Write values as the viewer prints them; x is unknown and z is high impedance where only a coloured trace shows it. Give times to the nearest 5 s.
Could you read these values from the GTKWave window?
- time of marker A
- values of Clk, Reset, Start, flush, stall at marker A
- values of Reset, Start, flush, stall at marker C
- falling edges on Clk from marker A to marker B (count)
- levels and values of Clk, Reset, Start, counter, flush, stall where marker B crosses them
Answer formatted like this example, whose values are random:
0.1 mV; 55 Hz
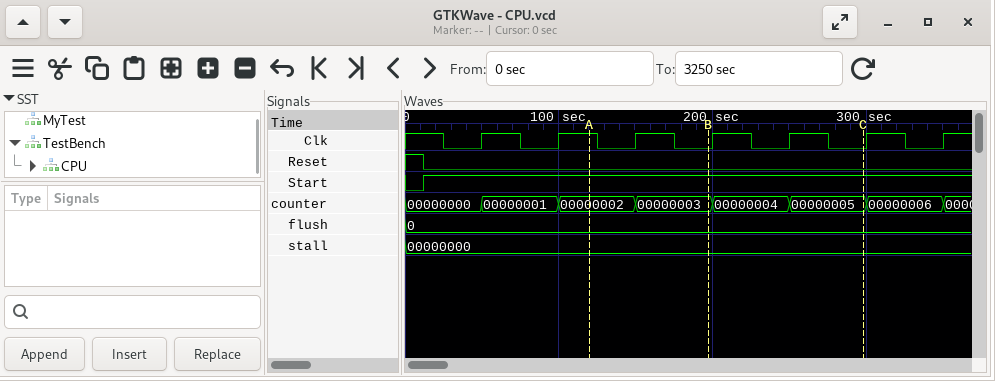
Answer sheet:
120 s; Clk=1, Reset=0, Start=1, flush=0, stall=00000000; Reset=0, Start=1, flush=0, stall=00000000; 2; Clk=0, Reset=0, Start=1, counter=00000003, flush=0, stall=00000000
